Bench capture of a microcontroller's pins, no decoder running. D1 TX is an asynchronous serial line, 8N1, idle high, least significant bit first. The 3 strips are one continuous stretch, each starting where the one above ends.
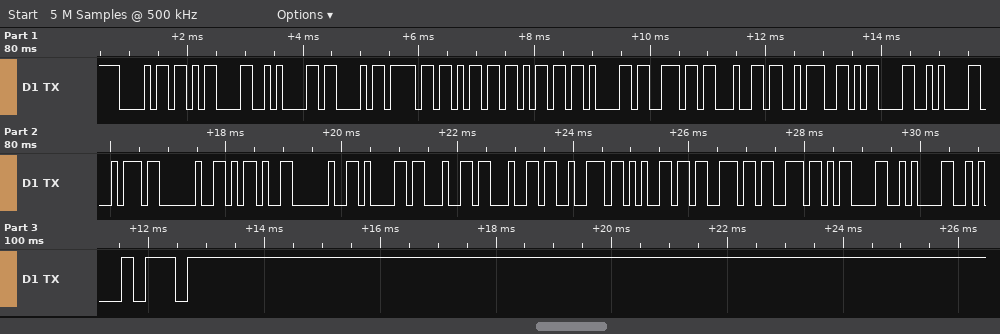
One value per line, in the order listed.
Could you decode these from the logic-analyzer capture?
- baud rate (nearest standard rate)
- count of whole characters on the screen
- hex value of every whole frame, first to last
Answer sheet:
9600 baud
28
0x68 0x0D 0x0A 0x43 0x6F 0x6D 0x6D 0x61 0x6E 0x64 0x3A 0x0D 0x0A 0x74 0x20 0x2D 0x20 0x61 0x64 0x64 0x72 0x65 0x73 0x73 0x0D 0x0A 0x0A 0x3E
